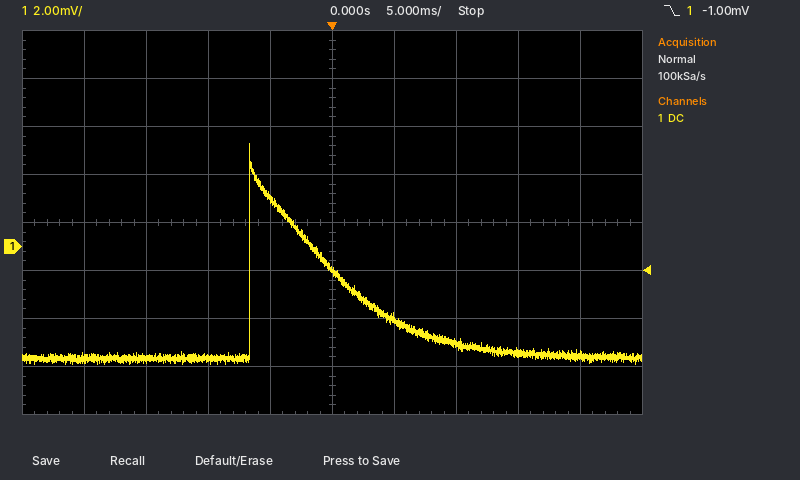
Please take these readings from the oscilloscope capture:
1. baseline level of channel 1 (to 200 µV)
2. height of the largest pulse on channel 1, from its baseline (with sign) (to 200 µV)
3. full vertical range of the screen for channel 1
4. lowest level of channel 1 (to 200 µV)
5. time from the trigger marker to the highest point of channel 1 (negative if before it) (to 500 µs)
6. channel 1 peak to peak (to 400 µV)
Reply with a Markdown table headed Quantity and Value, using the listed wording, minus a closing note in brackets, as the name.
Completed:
| Quantity | Value |
|---|---|
| baseline level of channel 1 | -4.6 mV |
| height of the largest pulse on channel 1, from its baseline (with sign) | +9.0 mV |
| full vertical range of the screen for channel 1 | 16 mV |
| lowest level of channel 1 | -5.0 mV |
| time from the trigger marker to the highest point of channel 1 (negative if before it) | -6.5 ms |
| channel 1 peak to peak | 9.2 mV |
